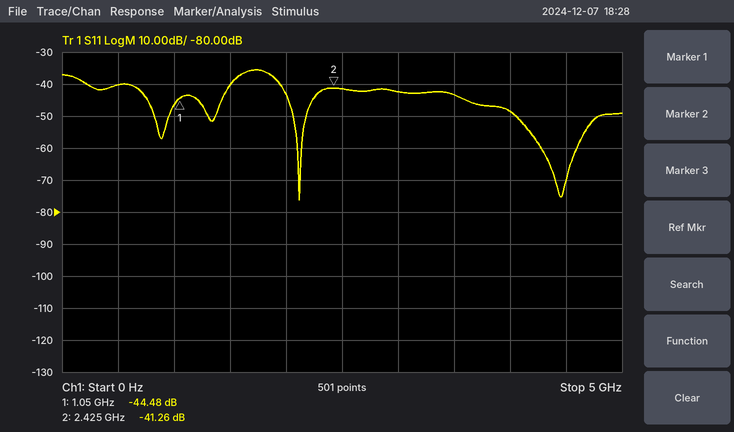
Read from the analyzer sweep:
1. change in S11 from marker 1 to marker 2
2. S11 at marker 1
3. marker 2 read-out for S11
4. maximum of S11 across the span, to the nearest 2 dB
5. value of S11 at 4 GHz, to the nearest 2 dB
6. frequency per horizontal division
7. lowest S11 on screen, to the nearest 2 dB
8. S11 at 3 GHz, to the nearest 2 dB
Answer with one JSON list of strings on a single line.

["3.22 dB", "-44.48 dB", "-41.26 dB", "-36 dB", "-48 dB", "500 MHz", "-76 dB", "-42 dB"]
